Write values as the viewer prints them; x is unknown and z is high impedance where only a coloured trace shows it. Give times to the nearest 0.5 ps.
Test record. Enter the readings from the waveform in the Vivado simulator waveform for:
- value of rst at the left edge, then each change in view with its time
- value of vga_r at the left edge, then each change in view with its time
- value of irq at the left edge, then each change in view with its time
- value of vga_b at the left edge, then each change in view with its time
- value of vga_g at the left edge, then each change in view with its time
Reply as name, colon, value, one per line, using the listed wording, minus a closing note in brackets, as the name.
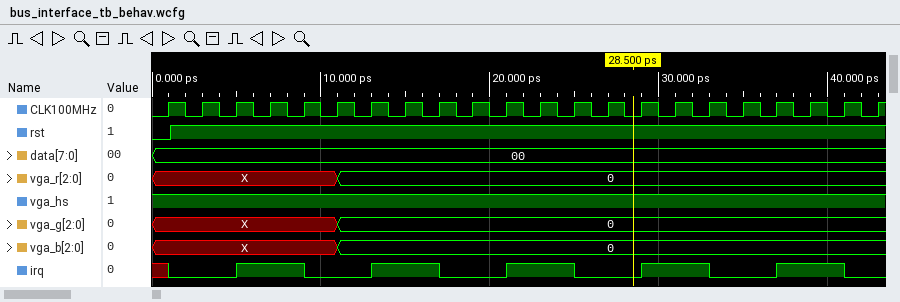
value of rst at the left edge, then each change in view with its time: 0, 1 at 1 ps
value of vga_r at the left edge, then each change in view with its time: X, 0 at 11 ps
value of irq at the left edge, then each change in view with its time: x, 0 at 1 ps, 1 at 5 ps, 0 at 9 ps, 1 at 13 ps, 0 at 17 ps, 1 at 21 ps, 0 at 25 ps, 1 at 29 ps, 0 at 33 ps, 1 at 37 ps, 0 at 41 ps
value of vga_b at the left edge, then each change in view with its time: X, 0 at 11 ps
value of vga_g at the left edge, then each change in view with its time: X, 0 at 11 ps
